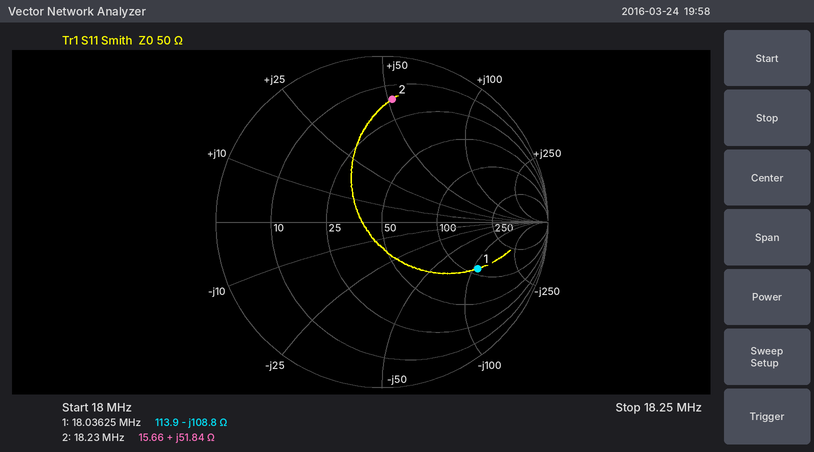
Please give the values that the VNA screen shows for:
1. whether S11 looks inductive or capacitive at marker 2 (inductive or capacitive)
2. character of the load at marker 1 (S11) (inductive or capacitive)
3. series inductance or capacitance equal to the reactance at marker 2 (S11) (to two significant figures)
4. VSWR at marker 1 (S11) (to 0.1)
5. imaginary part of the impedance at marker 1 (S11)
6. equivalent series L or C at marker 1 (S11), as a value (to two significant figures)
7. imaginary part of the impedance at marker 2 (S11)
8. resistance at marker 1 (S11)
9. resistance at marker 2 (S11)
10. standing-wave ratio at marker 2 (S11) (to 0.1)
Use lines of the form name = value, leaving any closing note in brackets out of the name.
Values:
whether S11 looks inductive or capacitive at marker 2 = inductive
character of the load at marker 1 (S11) = capacitive
series inductance or capacitance equal to the reactance at marker 2 (S11) = 450 nH
VSWR at marker 1 (S11) = 4.6
imaginary part of the impedance at marker 1 = -108.8 Ω
equivalent series L or C at marker 1 (S11), as a value = 81 pF
imaginary part of the impedance at marker 2 = +51.84 Ω
resistance at marker 1 = 113.9 Ω
resistance at marker 2 = 15.66 Ω
standing-wave ratio at marker 2 (S11) = 6.8
